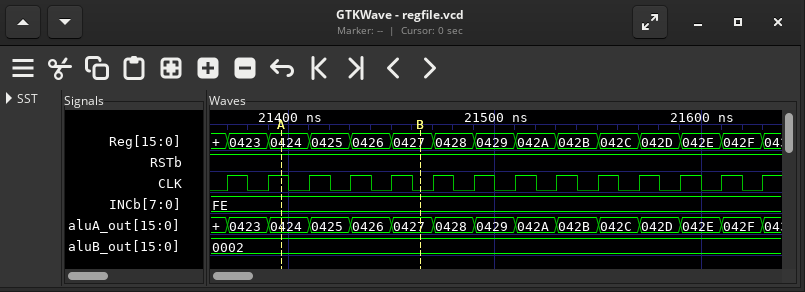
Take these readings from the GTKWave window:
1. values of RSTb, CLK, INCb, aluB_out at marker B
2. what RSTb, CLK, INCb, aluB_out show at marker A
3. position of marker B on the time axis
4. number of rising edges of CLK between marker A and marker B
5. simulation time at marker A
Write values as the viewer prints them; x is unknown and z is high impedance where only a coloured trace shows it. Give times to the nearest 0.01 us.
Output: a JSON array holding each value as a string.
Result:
["RSTb=1, CLK=0, INCb=FE, aluB_out=0002", "RSTb=1, CLK=1, INCb=FE, aluB_out=0002", "21.46 us", "3", "21.4 us"]
